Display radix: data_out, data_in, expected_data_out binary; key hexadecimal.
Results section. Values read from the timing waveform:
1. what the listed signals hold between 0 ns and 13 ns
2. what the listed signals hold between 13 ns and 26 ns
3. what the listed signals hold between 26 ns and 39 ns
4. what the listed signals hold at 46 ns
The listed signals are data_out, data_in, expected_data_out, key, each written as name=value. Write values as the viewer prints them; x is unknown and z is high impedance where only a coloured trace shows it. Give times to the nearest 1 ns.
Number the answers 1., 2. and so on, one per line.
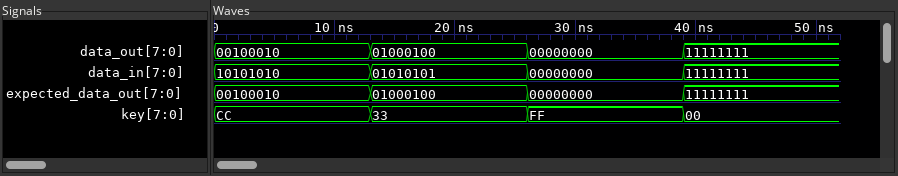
1. data_out=00100010, data_in=10101010, expected_data_out=00100010, key=CC
2. data_out=01000100, data_in=01010101, expected_data_out=01000100, key=33
3. data_out=00000000, data_in=00000000, expected_data_out=00000000, key=FF
4. data_out=11111111, data_in=11111111, expected_data_out=11111111, key=00
